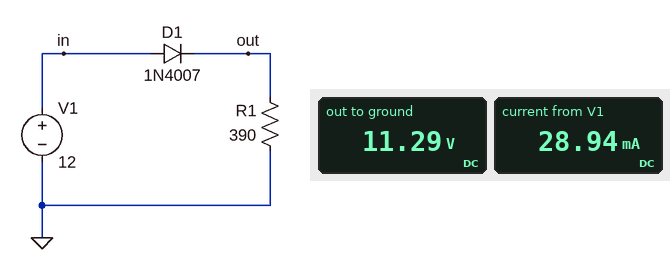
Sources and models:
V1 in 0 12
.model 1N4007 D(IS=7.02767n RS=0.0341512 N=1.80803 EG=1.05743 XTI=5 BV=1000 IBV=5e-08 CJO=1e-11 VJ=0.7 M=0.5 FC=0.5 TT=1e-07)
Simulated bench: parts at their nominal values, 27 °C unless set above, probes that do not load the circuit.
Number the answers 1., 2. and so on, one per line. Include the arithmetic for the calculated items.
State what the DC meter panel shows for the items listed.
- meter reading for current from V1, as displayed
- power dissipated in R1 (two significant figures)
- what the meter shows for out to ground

1. 28.94 mA
2. (11.29 V)^2 / 390 Ω = 330 mW
3. 11.29 V
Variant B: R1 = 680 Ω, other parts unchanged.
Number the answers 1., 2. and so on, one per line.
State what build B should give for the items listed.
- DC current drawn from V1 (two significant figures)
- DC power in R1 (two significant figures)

1. 17 mA
2. 190 mW
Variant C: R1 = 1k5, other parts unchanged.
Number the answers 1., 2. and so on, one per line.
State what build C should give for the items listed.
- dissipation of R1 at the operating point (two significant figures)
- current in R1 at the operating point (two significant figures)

1. 86 mW
2. 7.6 mA
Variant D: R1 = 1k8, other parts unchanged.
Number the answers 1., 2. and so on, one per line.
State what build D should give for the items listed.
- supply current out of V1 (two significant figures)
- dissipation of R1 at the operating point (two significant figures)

1. 6.3 mA
2. 72 mW
